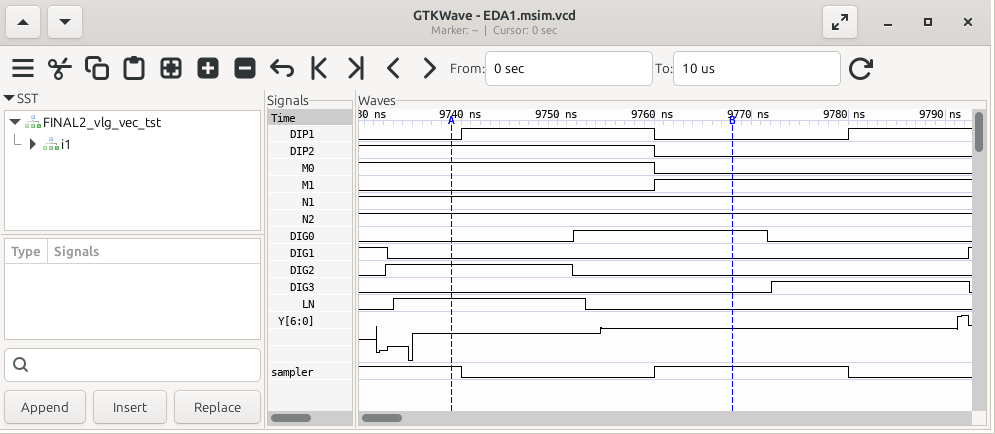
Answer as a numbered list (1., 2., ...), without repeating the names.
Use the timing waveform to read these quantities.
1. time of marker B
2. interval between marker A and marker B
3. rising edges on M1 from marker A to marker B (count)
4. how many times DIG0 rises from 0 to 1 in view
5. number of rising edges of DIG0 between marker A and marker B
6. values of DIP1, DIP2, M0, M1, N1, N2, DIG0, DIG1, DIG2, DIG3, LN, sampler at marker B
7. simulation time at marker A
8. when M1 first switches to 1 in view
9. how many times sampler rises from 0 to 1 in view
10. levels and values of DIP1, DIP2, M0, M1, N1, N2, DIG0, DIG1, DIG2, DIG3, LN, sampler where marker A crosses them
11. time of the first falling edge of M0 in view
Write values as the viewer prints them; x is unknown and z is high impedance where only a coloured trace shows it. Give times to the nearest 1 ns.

1. 9768 ns
2. 29 ns
3. 1
4. 1
5. 1
6. DIP1=0, DIP2=0, M0=0, M1=1, N1=1, N2=1, DIG0=1, DIG1=0, DIG2=0, DIG3=0, LN=0, sampler=1
7. 9739 ns
8. 9760 ns
9. 1
10. DIP1=0, DIP2=1, M0=1, M1=0, N1=1, N2=1, DIG0=0, DIG1=0, DIG2=1, DIG3=0, LN=1, sampler=1
11. 9760 ns
